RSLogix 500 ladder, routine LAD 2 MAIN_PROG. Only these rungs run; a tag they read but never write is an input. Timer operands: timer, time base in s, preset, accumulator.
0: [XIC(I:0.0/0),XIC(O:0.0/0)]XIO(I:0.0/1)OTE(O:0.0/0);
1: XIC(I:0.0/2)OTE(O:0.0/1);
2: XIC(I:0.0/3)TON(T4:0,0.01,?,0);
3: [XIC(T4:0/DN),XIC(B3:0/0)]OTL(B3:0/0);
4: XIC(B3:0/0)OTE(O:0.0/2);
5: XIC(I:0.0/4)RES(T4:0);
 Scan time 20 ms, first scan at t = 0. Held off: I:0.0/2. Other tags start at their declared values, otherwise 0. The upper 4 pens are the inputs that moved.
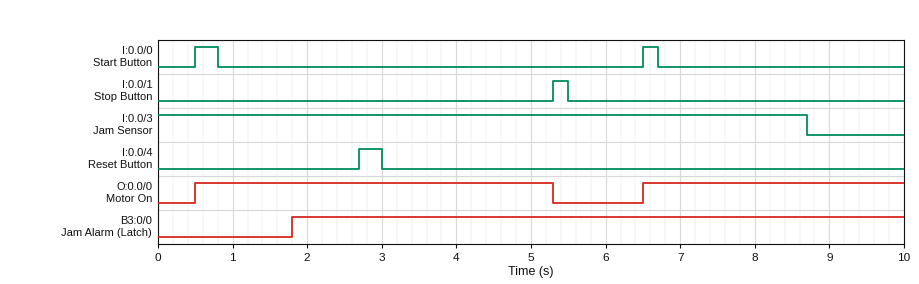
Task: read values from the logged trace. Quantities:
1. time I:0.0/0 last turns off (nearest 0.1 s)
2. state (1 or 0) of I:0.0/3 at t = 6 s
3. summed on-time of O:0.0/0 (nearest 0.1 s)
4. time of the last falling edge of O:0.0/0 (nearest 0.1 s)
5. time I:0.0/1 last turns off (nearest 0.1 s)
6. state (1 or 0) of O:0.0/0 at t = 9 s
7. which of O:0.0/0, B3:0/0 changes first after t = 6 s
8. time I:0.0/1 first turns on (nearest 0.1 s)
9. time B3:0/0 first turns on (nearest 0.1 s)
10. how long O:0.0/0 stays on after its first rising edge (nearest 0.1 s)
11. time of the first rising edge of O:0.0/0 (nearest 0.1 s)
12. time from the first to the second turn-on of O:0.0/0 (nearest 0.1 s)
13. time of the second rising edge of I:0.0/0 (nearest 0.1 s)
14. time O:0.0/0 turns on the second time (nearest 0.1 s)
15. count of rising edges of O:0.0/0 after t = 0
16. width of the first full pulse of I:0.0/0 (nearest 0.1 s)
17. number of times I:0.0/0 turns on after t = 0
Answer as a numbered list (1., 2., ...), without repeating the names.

1. 6.7 s
2. 1
3. 8.3 s
4. 5.3 s
5. 5.5 s
6. 1
7. O:0.0/0
8. 5.3 s
9. 1.8 s
10. 4.8 s
11. 0.5 s
12. 6.0 s
13. 6.5 s
14. 6.5 s
15. 2
16. 0.3 s
17. 2
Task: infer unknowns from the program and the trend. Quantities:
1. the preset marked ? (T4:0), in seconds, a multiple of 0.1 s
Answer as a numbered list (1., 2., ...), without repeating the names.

1. 1.8 s
